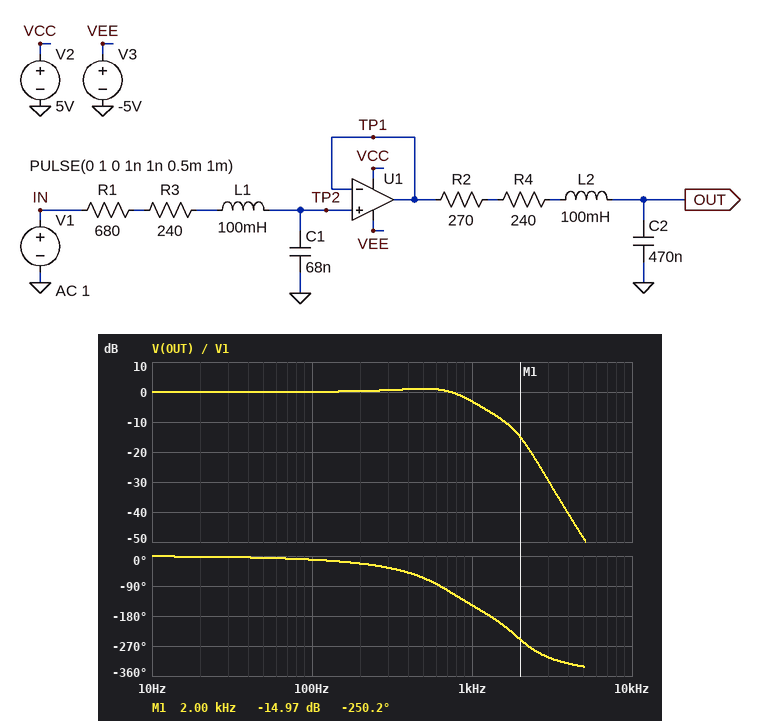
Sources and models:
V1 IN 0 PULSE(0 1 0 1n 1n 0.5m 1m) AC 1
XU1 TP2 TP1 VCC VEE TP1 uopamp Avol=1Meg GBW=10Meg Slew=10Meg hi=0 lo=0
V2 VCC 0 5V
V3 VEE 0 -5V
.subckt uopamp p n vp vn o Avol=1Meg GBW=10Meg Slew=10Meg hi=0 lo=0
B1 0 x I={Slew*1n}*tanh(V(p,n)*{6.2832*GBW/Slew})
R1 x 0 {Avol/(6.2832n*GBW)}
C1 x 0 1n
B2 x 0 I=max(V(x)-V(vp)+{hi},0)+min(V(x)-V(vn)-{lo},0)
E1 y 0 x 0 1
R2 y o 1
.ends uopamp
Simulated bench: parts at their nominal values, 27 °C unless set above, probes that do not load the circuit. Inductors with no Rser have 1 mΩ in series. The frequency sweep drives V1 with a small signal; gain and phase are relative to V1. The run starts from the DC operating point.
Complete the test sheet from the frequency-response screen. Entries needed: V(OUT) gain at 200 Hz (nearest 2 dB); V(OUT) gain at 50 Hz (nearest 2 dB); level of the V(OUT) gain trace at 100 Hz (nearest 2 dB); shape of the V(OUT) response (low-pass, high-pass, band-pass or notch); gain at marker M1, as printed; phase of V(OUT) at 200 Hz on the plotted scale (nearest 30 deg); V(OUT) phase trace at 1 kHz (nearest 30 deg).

0 dB
0 dB
0 dB
low-pass
-14.97 dB
-30 deg
-150 deg
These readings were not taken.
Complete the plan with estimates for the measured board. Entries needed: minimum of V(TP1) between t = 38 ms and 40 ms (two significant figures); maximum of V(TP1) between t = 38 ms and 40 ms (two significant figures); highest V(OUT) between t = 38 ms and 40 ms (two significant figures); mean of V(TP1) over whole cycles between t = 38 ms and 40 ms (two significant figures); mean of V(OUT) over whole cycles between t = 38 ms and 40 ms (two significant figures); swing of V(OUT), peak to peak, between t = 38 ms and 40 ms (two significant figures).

-260 mV
1.3 V
950 mV
500 mV
500 mV
900 mV
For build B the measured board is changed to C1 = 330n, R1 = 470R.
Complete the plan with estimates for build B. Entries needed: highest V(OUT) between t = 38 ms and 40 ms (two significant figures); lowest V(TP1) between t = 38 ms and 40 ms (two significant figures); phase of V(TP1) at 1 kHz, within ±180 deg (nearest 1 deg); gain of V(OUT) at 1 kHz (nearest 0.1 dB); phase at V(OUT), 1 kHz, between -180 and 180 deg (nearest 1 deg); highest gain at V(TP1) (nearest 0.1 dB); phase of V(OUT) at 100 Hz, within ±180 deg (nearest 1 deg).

740 mV
55 mV
-102 deg
-8.3 dB
139 deg
0.1 dB
-17 deg
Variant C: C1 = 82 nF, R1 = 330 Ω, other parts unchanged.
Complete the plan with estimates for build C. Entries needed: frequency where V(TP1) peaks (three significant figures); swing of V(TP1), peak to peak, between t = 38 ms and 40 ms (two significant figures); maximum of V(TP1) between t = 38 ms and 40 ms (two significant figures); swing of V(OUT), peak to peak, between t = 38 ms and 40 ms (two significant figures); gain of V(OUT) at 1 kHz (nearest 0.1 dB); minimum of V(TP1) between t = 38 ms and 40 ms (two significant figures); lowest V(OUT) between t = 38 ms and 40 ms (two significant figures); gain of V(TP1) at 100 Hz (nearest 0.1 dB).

1.64 kHz
1.8 V
1.4 V
1.0 V
-2.1 dB
-390 mV
-1.2 mV
0 dB
